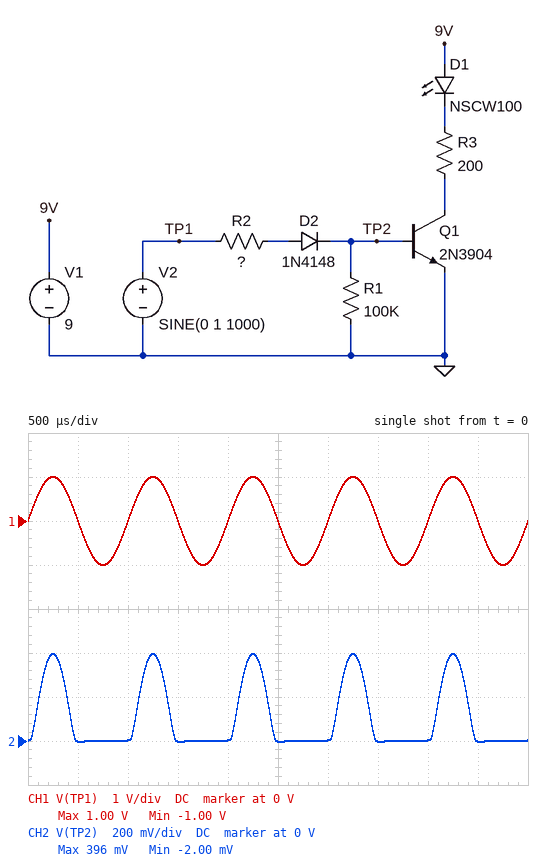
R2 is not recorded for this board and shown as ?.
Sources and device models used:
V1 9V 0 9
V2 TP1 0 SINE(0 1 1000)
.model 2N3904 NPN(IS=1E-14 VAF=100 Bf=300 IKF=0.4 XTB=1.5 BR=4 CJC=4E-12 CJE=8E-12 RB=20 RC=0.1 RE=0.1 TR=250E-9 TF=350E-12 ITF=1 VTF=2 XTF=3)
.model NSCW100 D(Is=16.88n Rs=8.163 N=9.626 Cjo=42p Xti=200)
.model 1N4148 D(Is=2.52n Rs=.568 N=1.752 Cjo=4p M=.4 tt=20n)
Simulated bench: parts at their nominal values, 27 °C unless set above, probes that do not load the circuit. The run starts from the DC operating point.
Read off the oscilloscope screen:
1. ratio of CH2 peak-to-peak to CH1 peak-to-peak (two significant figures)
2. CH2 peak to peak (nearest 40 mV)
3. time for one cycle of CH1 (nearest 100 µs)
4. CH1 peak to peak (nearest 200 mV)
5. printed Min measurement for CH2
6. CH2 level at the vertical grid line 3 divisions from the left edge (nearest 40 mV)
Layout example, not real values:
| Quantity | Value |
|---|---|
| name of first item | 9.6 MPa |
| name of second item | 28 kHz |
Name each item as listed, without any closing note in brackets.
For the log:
| Quantity | Value |
|---|---|
| ratio of CH2 peak-to-peak to CH1 peak-to-peak | 0.20 |
| CH2 peak to peak | 400 mV |
| time for one cycle of CH1 | 1.0 ms |
| CH1 peak to peak | 2.0 V |
| printed Min measurement for CH2 | -2.00 mV |
| CH2 level at the vertical grid line 3 divisions from the left edge | 0 V |
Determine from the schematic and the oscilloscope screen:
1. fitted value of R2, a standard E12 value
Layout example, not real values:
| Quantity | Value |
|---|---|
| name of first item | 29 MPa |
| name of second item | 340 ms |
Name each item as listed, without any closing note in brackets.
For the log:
| Quantity | Value |
|---|---|
| fitted value of R2, a standard E12 value | 68 kΩ |
